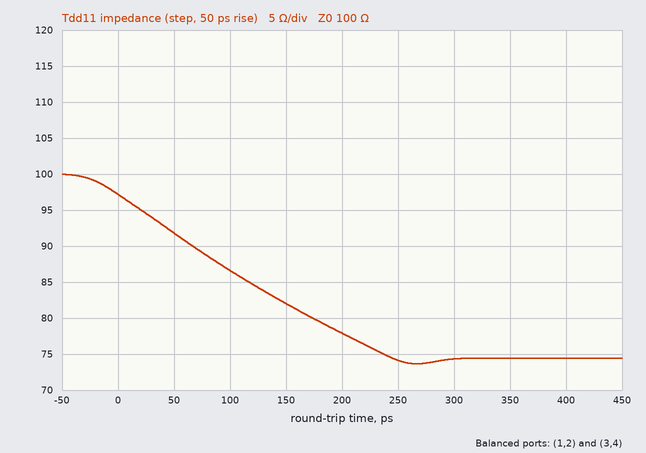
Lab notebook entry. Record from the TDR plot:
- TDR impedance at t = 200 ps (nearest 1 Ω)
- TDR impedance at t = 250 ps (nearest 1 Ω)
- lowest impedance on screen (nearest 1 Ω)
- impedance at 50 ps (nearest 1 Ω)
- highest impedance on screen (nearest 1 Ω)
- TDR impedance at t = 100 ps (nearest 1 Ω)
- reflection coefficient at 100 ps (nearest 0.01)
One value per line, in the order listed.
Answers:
78 Ω
74 Ω
74 Ω
92 Ω
100 Ω
87 Ω
-0.07
